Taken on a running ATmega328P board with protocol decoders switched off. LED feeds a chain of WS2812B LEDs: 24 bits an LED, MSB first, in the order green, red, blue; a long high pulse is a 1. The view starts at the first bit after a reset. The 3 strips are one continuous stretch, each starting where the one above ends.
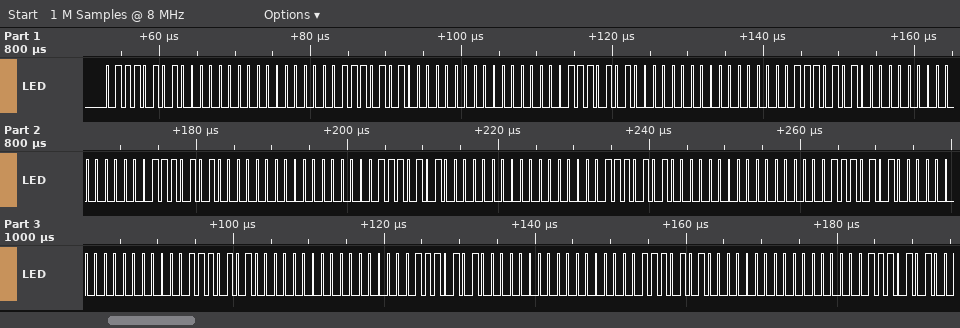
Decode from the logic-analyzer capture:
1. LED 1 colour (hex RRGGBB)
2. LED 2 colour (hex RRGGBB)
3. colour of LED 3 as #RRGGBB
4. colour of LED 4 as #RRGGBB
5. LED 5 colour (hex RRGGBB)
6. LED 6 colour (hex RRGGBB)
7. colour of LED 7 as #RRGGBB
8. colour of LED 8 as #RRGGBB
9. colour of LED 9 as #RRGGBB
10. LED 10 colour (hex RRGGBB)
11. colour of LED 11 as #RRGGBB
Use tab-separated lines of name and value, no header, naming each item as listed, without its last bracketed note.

LED 1 colour	#007500
LED 2 colour	#007500
colour of LED 3 as #RRGGBB	#007500
colour of LED 4 as #RRGGBB	#007500
LED 5 colour	#007500
LED 6 colour	#007500
colour of LED 7 as #RRGGBB	#007500
colour of LED 8 as #RRGGBB	#007500
colour of LED 9 as #RRGGBB	#007500
LED 10 colour	#007500
colour of LED 11 as #RRGGBB	#007500
